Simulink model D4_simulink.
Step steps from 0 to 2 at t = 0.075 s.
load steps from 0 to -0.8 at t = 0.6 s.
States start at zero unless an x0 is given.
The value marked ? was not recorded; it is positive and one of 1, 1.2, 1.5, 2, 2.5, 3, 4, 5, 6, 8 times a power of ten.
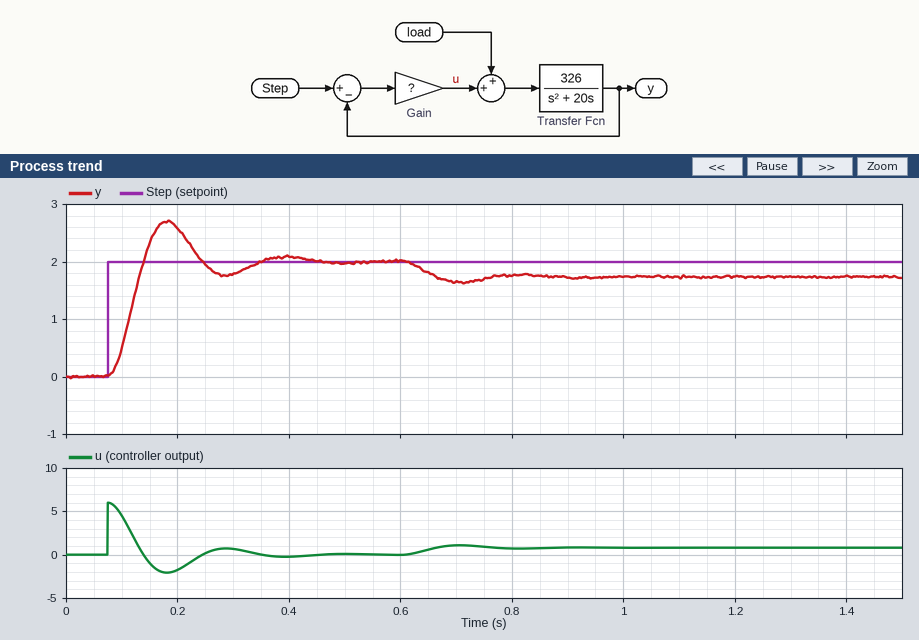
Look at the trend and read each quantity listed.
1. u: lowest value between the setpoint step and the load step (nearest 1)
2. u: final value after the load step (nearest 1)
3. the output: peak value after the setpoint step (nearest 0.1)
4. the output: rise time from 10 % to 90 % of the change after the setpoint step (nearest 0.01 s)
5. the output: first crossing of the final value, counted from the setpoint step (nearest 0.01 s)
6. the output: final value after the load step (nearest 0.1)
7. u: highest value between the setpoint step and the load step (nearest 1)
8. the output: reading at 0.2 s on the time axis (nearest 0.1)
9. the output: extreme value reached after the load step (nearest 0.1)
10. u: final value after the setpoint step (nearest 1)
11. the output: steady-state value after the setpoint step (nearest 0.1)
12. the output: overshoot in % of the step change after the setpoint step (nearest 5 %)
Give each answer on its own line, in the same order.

-2
1
2.7
0.04 s
0.06 s
1.7
6
2.6
1.6
0
2.0
35 %
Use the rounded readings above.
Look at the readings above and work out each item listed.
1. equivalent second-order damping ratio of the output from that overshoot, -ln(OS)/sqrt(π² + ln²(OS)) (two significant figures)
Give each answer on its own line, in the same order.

0.32
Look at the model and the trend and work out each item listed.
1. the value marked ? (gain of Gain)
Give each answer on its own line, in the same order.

3
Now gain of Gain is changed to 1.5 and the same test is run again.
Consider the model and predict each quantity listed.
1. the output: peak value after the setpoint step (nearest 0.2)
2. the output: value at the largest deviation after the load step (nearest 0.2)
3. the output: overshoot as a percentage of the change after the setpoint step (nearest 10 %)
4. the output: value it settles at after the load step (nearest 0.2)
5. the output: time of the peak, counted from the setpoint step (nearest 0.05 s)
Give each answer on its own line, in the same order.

2.4
1.4
20 %
1.4
0.15 s
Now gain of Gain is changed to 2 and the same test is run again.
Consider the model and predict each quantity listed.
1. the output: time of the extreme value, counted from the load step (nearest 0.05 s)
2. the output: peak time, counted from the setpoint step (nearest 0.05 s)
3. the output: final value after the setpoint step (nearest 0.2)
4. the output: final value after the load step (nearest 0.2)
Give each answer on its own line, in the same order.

0.15 s
0.15 s
2.0
1.6
